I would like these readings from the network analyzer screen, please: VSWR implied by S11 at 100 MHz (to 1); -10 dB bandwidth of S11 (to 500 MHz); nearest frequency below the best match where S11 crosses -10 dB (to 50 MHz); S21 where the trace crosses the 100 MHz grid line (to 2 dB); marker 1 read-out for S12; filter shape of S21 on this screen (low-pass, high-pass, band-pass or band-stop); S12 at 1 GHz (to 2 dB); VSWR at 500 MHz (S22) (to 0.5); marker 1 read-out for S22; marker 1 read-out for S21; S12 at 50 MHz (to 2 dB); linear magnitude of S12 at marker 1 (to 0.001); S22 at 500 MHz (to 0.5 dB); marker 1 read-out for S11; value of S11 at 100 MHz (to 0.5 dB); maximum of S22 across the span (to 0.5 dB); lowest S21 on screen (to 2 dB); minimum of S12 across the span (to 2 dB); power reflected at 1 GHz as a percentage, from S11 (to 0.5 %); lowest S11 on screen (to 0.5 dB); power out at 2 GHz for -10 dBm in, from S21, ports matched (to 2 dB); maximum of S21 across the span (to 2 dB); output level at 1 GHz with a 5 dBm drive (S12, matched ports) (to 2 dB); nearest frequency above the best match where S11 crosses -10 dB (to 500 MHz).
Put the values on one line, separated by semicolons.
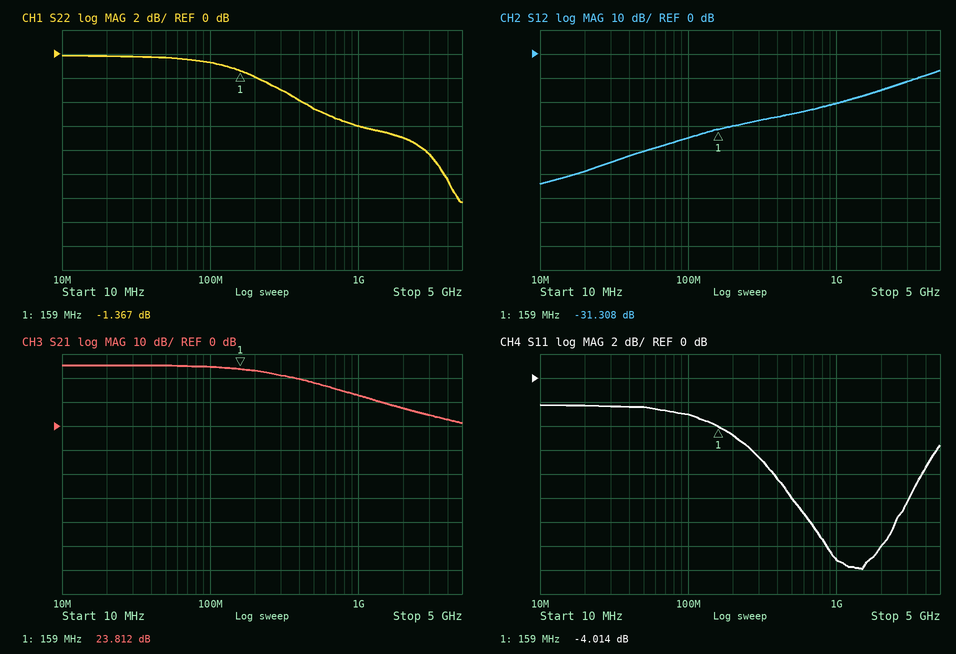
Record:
6; 2.5 GHz; 500 MHz; 24 dB; -31.308 dB; low-pass; -20 dB; 4.0; -1.367 dB; 23.812 dB; -40 dB; 0.027; -4.5 dB; -4.014 dB; -3.0 dB; 0.0 dB; 2 dB; -54 dB; 3.0 %; -16.0 dB; -2 dBm; 26 dB; -16 dBm; 3.0 GHz
